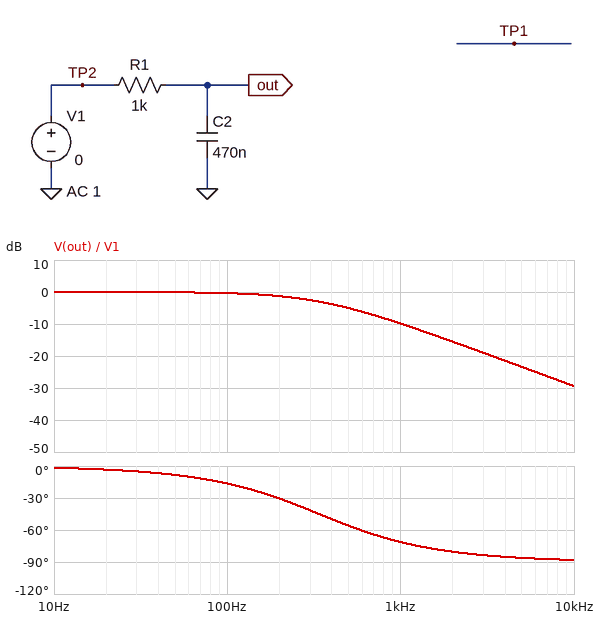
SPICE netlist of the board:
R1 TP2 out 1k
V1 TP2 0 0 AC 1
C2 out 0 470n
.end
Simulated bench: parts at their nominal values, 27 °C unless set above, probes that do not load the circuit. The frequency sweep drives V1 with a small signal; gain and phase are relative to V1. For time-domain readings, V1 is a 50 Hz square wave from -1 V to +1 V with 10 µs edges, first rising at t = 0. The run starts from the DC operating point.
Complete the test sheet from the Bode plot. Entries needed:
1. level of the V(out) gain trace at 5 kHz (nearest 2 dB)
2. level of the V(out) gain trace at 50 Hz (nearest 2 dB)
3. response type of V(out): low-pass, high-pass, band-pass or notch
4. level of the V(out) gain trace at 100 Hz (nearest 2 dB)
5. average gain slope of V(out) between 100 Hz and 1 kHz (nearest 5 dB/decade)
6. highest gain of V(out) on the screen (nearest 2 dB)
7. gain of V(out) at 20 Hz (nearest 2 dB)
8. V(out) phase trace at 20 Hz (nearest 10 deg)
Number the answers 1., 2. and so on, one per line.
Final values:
1. -24 dB
2. 0 dB
3. low-pass
4. 0 dB
5. -10 dB/decade
6. 0 dB
7. 0 dB
8. 0 deg
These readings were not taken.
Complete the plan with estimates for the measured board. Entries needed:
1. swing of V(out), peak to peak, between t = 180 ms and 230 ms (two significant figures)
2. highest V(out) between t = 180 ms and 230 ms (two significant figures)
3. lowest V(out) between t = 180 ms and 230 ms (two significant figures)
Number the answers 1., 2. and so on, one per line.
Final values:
1. 2.0 V
2. 1.0 V
3. -1.0 V
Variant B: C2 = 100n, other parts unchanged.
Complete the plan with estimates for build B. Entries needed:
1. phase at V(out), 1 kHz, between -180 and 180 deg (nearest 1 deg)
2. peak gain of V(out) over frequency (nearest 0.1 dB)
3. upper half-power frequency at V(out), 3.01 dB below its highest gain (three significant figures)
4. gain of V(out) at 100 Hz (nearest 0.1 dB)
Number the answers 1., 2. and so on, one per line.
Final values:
1. -32 deg
2. 0 dB
3. 1.59 kHz
4. 0 dB
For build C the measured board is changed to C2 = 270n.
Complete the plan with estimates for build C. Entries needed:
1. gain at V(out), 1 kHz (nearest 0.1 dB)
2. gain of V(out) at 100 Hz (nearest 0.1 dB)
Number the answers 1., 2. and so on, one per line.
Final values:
1. -5.9 dB
2. -0.1 dB
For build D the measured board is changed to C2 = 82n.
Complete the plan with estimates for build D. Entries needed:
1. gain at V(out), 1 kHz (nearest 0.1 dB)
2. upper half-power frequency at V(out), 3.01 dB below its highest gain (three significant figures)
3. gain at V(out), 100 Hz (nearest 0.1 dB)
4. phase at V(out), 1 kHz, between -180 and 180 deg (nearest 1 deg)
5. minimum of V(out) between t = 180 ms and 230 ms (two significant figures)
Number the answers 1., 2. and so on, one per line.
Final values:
1. -1.0 dB
2. 1.94 kHz
3. 0 dB
4. -27 deg
5. -1.0 V
